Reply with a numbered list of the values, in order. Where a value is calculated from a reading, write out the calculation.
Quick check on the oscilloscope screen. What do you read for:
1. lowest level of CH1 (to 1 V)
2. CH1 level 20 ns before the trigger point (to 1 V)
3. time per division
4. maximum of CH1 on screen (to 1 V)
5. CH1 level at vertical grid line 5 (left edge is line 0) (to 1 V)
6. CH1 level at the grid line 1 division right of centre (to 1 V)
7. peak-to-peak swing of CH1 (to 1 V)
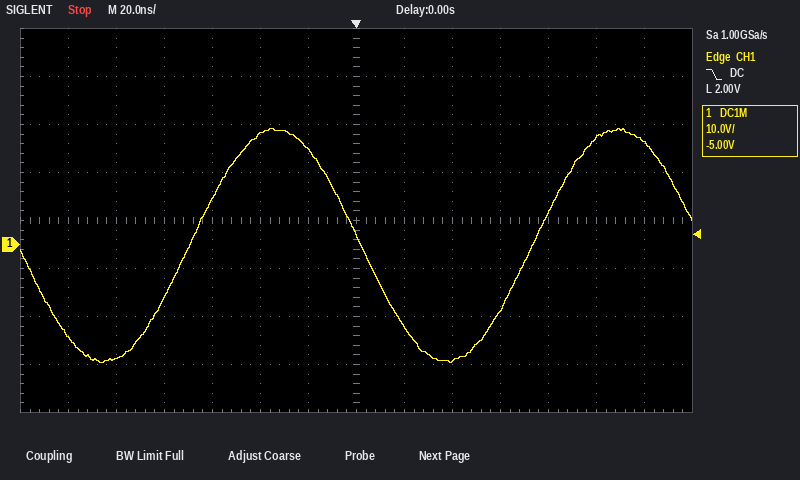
1. -25 V
2. 20 V
3. 20 ns
4. 24 V
5. 23 V
6. -17 V
7. 24 V − (-25 V) = 49 V
